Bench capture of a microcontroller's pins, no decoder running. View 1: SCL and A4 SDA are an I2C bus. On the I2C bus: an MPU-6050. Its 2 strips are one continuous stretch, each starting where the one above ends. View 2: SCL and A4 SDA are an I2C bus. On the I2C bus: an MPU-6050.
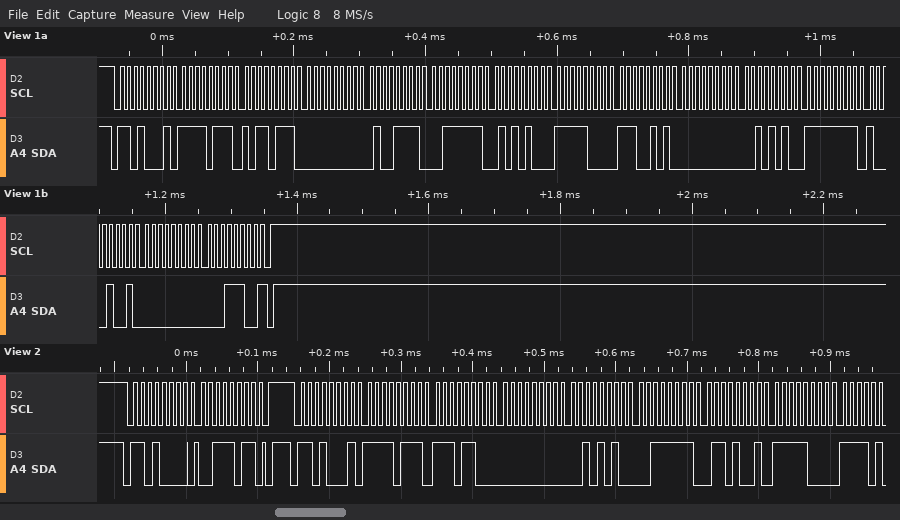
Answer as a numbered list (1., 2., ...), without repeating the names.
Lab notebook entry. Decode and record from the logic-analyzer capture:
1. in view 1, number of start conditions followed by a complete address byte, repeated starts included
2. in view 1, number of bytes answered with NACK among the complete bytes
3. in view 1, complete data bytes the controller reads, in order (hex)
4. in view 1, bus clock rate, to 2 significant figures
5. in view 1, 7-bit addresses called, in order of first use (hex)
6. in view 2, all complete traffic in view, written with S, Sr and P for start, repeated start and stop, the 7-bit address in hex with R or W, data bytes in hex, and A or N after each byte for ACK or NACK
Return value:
1. 1
2. 1
3. F7 B7 00 4F 3F 54 F8 E5 00 2A FF 89 00 1C
4. 100 kHz
5. 0x68
6. S 68W A 3B A P S 68R A F7 A EC A 00 A 2A A 3F A 69 A F8 A
